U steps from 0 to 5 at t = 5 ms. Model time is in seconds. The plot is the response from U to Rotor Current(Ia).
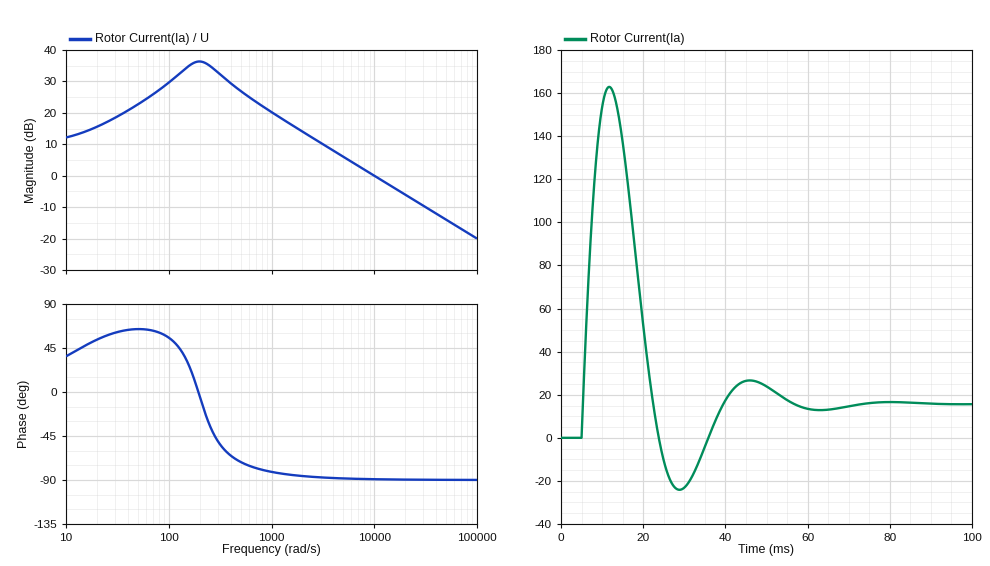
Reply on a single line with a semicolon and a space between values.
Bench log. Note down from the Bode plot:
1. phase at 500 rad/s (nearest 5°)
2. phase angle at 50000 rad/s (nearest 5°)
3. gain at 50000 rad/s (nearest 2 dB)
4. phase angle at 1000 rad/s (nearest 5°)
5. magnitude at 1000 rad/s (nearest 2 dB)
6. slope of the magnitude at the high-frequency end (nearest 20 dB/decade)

-70°; -90°; -14 dB; -80°; 20 dB; -20 dB/decade
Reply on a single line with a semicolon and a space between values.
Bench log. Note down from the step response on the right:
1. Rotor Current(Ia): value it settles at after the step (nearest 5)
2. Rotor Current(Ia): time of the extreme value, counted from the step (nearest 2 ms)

15; 6 ms
